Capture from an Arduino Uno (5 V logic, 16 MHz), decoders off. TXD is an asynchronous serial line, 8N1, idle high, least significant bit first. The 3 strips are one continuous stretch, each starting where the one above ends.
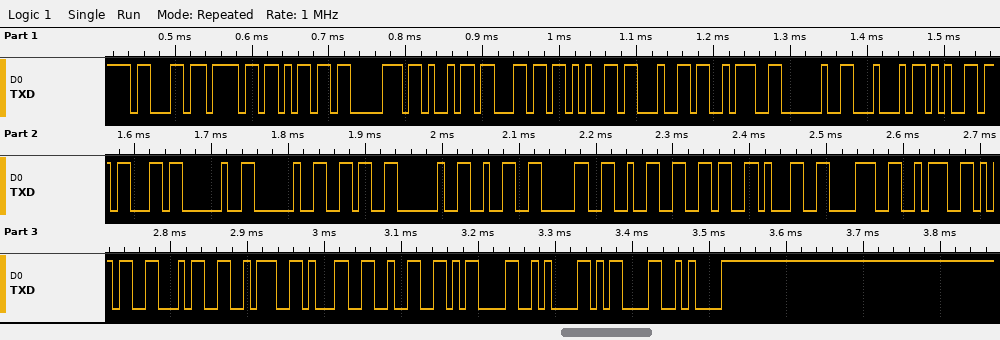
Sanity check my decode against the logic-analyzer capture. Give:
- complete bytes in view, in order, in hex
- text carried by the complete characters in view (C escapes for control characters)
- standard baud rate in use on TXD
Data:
63 6F 6D 70 69 6C 65 64 3A 20 44 65 63 20 20 36 20 32 30 32 36 31 38 3A 35 34 3A 31 32 0D 0A 0D 0A
"compiled: Dec  6 202618:54:12\r\n\r\n"
115200 baud
